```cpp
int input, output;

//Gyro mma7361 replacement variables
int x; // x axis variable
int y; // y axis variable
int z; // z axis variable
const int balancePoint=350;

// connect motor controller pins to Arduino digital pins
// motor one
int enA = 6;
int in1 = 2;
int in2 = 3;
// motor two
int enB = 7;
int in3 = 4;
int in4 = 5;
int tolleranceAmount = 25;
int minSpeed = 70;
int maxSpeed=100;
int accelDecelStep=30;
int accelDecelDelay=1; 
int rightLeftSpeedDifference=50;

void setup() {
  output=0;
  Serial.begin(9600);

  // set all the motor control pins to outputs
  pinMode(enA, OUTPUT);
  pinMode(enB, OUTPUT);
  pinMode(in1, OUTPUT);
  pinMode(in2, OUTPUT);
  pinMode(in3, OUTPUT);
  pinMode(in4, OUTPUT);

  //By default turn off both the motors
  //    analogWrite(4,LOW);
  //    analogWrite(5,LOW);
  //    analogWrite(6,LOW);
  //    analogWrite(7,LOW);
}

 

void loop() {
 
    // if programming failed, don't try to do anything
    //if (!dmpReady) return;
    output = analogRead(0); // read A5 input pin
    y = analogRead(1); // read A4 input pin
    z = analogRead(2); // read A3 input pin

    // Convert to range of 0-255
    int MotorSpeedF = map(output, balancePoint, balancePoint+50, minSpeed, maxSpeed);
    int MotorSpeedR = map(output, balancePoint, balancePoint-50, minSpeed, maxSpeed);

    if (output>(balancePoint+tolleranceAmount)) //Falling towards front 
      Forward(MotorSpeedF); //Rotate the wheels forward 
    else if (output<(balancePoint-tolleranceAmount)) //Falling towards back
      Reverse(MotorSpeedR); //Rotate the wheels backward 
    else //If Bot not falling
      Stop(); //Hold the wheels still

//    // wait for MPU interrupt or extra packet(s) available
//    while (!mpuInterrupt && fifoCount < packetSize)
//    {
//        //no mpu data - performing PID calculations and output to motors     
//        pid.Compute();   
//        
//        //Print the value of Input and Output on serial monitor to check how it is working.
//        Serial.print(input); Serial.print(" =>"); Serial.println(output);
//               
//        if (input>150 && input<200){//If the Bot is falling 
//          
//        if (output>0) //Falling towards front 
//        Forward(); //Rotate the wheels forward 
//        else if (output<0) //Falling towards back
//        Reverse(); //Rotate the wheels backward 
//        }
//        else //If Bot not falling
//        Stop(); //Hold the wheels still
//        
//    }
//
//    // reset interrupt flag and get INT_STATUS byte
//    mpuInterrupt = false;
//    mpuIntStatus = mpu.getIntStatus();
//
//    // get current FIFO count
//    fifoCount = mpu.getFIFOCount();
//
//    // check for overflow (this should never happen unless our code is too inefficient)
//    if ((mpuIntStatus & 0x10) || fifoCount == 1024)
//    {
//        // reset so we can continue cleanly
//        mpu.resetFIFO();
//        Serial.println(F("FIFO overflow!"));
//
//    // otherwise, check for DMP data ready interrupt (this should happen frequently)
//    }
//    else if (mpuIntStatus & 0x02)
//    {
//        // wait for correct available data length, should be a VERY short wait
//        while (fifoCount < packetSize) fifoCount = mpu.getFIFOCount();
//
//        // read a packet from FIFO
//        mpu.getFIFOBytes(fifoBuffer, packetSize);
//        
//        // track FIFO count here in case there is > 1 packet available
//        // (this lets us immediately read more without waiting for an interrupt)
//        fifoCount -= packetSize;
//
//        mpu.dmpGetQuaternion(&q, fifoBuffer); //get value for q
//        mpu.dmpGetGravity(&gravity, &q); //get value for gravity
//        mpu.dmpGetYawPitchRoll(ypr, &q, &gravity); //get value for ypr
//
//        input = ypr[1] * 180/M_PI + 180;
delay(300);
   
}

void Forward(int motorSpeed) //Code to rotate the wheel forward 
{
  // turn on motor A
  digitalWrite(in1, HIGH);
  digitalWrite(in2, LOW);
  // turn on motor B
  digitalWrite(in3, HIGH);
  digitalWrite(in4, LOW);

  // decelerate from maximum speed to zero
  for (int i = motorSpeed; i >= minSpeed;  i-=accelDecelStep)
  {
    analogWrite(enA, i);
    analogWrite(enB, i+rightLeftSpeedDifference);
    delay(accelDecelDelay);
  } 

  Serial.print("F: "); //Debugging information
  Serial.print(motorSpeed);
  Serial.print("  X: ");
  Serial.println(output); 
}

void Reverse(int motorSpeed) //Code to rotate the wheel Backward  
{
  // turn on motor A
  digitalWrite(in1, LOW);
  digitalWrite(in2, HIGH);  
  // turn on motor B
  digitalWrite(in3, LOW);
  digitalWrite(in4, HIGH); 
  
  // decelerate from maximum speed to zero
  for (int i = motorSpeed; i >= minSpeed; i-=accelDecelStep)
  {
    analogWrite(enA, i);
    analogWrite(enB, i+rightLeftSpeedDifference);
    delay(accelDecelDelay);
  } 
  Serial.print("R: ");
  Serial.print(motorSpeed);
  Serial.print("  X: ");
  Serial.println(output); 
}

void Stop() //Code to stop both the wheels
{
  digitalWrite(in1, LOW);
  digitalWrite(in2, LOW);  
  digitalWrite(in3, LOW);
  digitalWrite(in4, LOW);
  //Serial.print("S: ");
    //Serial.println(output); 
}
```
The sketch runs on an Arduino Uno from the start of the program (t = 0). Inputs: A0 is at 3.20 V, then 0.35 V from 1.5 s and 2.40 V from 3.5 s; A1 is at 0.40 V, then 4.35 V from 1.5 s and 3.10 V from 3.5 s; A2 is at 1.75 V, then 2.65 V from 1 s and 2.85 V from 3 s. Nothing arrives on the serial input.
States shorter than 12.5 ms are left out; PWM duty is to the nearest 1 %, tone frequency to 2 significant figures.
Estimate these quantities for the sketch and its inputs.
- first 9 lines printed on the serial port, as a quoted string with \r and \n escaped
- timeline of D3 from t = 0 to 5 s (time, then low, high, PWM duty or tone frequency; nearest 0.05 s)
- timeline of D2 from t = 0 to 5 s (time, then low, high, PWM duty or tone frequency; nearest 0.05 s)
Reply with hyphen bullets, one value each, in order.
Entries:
- "F: 253  X: 655\r\nF: 253  X: 655\r\nF: 253  X: 655\r\nF: 253  X: 655\r\nF: 253  X: 655\r\nR: 237  X: 71\r\nR: 237  X: 71\r\nR: 237  X: 71\r\nR: 237  X: 71\r\n"
- 0 s low; 1.55 s high; 3.7 s low
- 0 s high; 1.55 s low; 3.7 s high
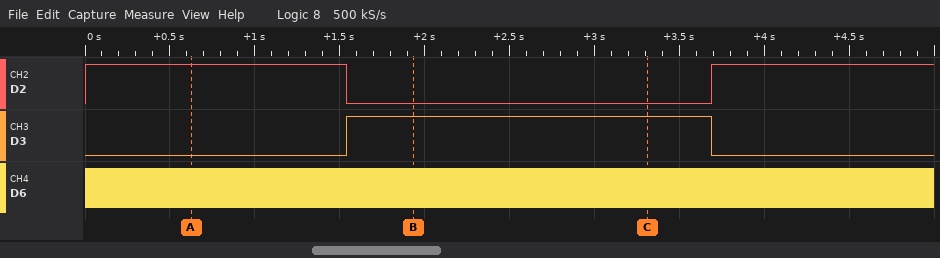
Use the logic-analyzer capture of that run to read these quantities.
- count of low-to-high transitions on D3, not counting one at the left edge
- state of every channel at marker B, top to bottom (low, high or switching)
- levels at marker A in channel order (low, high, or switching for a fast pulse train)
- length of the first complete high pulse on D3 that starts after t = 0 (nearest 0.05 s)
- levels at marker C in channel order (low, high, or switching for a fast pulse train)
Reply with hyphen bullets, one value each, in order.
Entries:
- 1
- D2 low, D3 high, D6 switching
- D2 high, D3 low, D6 switching
- 2.15 s
- D2 low, D3 high, D6 switching
